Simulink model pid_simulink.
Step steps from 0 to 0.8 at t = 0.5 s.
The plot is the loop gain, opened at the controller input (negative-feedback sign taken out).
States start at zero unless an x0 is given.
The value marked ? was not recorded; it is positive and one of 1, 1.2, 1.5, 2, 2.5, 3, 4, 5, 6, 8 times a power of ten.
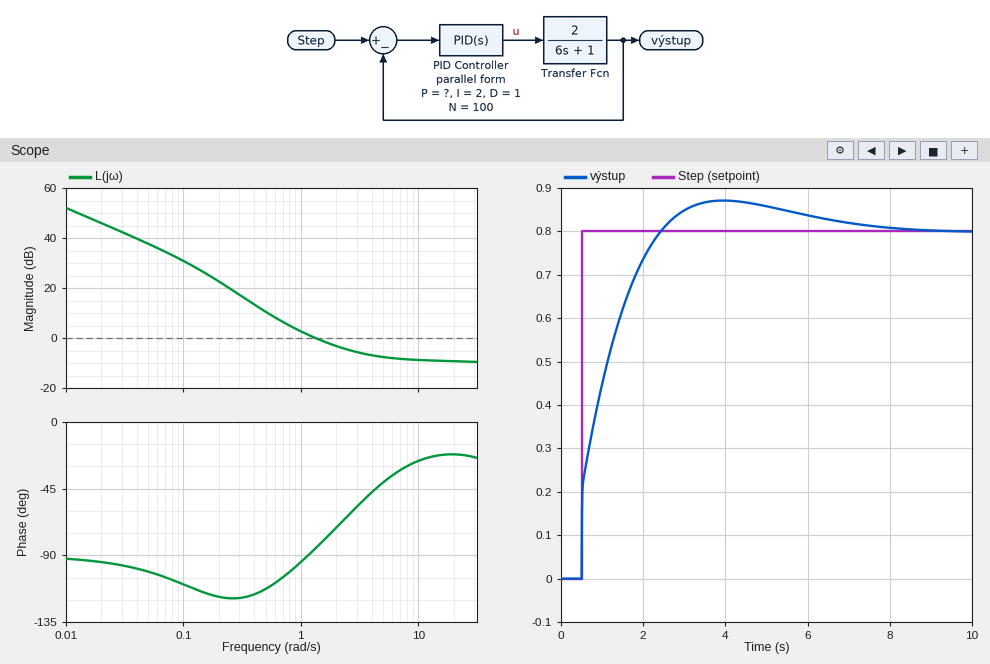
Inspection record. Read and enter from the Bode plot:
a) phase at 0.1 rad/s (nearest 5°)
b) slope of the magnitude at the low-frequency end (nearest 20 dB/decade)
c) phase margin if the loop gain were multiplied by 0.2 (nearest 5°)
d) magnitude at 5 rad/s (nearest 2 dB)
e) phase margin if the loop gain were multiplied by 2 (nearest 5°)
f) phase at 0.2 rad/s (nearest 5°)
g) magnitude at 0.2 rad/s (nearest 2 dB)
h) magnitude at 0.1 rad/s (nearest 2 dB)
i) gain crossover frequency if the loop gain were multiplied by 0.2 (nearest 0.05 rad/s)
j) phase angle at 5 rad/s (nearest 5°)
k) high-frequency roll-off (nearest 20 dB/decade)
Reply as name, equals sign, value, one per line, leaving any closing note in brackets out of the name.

phase at 0.1 rad/s = -110°
slope of the magnitude at the low-frequency end = -20 dB/decade
phase margin if the loop gain were multiplied by 0.2 = 65°
magnitude at 5 rad/s = -8 dB
phase margin if the loop gain were multiplied by 2 = 125°
phase at 0.2 rad/s = -120°
magnitude at 0.2 rad/s = 22 dB
magnitude at 0.1 rad/s = 30 dB
gain crossover frequency if the loop gain were multiplied by 0.2 = 0.40 rad/s
phase angle at 5 rad/s = -40°
high-frequency roll-off = 0 dB/decade
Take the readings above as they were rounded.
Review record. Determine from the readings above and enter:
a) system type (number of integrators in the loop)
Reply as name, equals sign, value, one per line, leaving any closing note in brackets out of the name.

system type = 1
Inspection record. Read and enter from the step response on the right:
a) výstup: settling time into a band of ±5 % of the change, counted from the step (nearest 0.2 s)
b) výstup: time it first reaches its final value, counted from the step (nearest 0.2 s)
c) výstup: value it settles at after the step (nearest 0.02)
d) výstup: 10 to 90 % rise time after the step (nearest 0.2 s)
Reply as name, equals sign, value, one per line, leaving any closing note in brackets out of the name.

výstup: settling time into a band of ±5 % of the change, counted from the step = 5.4 s
výstup: time it first reaches its final value, counted from the step = 2.0 s
výstup: value it settles at after the step = 0.80
výstup: 10 to 90 % rise time after the step = 1.4 s
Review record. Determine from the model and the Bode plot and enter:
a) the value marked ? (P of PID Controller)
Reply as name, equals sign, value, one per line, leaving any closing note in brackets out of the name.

the value marked ? = 4
